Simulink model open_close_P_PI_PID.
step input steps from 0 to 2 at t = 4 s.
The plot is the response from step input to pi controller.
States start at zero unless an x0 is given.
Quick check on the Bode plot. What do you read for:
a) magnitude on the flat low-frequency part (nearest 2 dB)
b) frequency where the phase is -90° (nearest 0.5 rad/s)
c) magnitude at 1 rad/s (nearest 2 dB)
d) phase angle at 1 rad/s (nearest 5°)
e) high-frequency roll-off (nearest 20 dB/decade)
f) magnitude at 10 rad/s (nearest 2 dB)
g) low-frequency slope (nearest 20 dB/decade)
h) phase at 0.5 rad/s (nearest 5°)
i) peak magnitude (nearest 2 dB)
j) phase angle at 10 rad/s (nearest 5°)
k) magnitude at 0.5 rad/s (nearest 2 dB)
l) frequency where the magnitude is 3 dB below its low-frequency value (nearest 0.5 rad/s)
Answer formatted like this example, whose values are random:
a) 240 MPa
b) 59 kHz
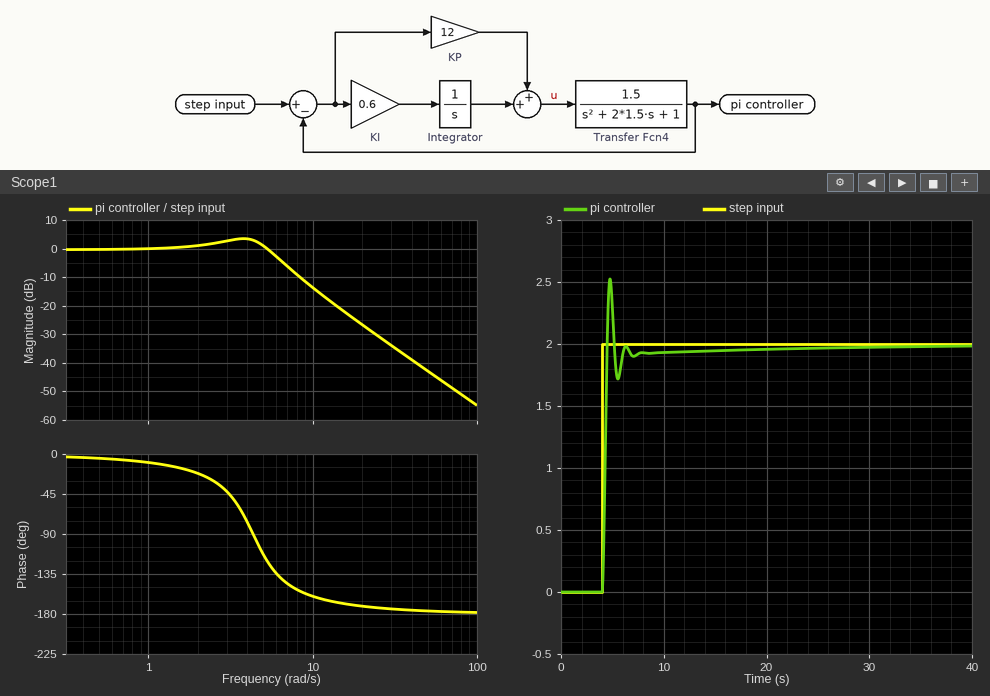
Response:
a) 0 dB
b) 4.5 rad/s
c) 0 dB
d) -10°
e) -40 dB/decade
f) -14 dB
g) 0 dB/decade
h) -5°
i) 4 dB
j) -160°
k) 0 dB
l) 6.0 rad/s
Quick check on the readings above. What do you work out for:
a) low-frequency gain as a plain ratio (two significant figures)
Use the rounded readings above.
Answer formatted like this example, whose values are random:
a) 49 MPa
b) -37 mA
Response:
a) 1.0
